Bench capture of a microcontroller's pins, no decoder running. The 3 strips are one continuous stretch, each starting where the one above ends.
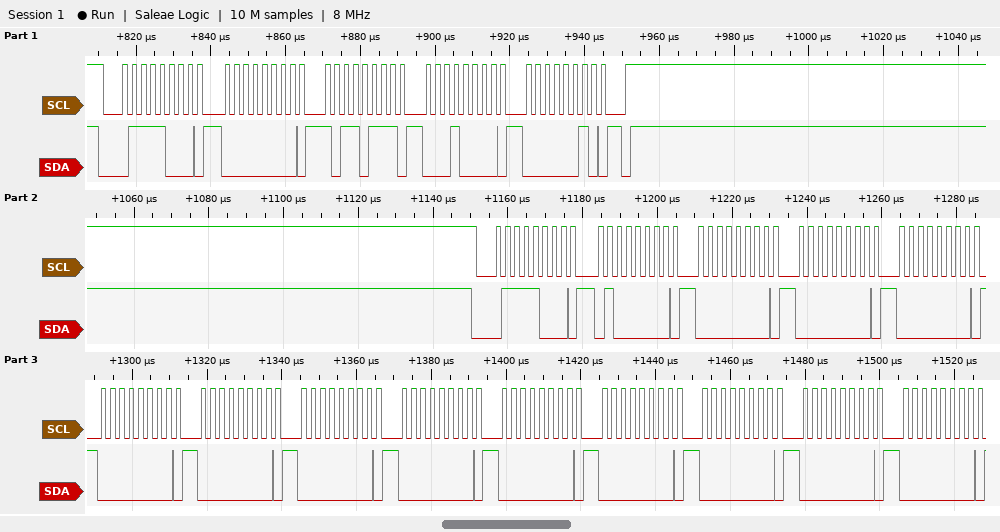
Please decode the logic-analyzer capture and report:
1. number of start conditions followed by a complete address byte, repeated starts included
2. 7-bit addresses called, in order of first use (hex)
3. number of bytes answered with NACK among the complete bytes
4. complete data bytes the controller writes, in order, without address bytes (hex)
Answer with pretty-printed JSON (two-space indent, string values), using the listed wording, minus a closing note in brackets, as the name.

{
  "number of start conditions followed by a complete address byte, repeated starts included": "2",
  "7-bit addresses called, in order of first use": "0x3C",
  "number of bytes answered with NACK among the complete bytes": "0",
  "complete data bytes the controller writes, in order, without address bytes": "00 B7 10 02 40 00 00 00 00 00 00 00 00 00 00 00 00"
}
